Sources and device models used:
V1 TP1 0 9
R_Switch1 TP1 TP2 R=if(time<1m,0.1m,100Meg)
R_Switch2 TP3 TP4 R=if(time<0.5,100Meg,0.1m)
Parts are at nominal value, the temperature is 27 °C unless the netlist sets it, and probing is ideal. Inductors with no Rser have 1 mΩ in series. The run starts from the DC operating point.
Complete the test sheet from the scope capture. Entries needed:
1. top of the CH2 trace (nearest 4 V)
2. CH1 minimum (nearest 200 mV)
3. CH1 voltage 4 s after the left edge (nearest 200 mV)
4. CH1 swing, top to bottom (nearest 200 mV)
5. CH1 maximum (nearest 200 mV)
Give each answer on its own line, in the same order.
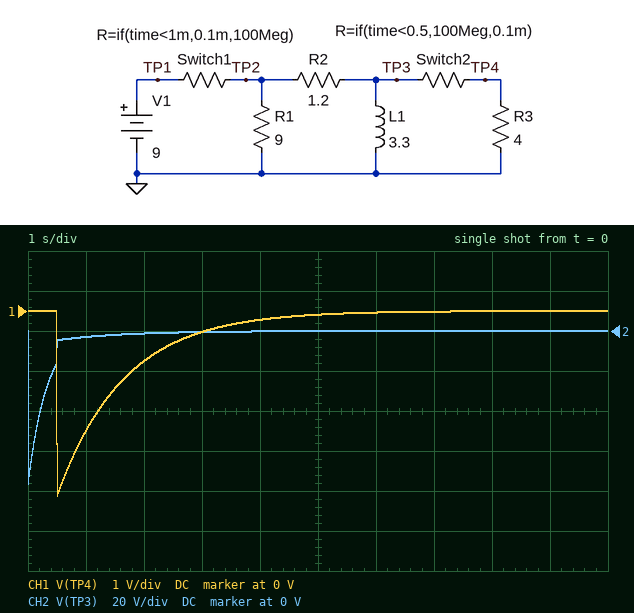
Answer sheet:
0 V
-4.6 V
-200 mV
4.6 V
0 V
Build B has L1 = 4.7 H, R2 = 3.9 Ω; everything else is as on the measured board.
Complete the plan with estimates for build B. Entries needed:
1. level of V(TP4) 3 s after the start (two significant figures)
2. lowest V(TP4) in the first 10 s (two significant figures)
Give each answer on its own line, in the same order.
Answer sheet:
-350 mV
-1.8 V
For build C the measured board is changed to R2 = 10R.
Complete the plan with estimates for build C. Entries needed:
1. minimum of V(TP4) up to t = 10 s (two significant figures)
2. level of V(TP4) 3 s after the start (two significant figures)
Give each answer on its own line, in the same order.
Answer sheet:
-170 mV
-14 mV
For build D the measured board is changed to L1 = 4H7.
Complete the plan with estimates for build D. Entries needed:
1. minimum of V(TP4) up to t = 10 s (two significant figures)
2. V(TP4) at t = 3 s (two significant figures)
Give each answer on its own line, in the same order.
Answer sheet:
-7.3 V
-1.6 V
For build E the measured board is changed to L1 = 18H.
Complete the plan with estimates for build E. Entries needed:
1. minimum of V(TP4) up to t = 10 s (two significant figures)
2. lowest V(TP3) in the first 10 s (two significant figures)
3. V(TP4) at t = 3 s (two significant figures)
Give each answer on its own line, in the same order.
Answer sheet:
-16 V
-76 V
-11 V
